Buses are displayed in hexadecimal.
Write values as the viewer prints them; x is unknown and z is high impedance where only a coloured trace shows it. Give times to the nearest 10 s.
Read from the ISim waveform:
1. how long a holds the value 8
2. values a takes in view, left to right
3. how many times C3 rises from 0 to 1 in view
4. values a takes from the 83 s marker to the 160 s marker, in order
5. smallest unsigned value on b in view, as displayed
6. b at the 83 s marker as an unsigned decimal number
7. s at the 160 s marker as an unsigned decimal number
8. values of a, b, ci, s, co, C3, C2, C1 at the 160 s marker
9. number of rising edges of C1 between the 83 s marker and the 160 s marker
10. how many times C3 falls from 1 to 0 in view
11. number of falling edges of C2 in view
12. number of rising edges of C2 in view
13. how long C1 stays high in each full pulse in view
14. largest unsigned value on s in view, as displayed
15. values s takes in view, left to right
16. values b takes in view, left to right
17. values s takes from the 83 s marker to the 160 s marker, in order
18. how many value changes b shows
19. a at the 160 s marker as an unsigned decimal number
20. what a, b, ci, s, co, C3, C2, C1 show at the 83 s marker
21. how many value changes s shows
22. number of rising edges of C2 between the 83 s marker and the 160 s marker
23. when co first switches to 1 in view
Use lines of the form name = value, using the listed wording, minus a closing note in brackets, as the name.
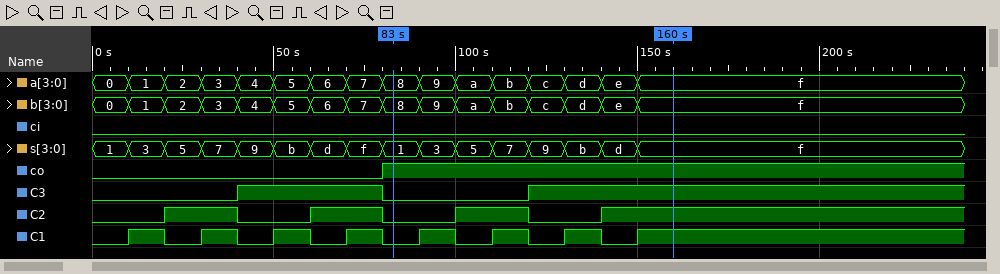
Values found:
how long a holds the value 8 = 10 s
values a takes in view, left to right = 0, 1, 2, 3, 4, 5, 6, 7, 8, 9, a, b, c, d, e, f
how many times C3 rises from 0 to 1 in view = 2
values a takes from the 83 s marker to the 160 s marker, in order = 8, 9, a, b, c, d, e, f
smallest unsigned value on b in view, as displayed = 0
b at the 83 s marker as an unsigned decimal number = 8
s at the 160 s marker as an unsigned decimal number = 15
values of a, b, ci, s, co, C3, C2, C1 at the 160 s marker = a=f, b=f, ci=0, s=f, co=1, C3=1, C2=1, C1=1
number of rising edges of C1 between the 83 s marker and the 160 s marker = 4
how many times C3 falls from 1 to 0 in view = 1
number of falling edges of C2 in view = 3
number of rising edges of C2 in view = 4
how long C1 stays high in each full pulse in view = 10 s, 10 s, 10 s, 10 s, 10 s, 10 s, 10 s
largest unsigned value on s in view, as displayed = f
values s takes in view, left to right = 1, 3, 5, 7, 9, b, d, f, 1, 3, 5, 7, 9, b, d, f
values b takes in view, left to right = 0, 1, 2, 3, 4, 5, 6, 7, 8, 9, a, b, c, d, e, f
values s takes from the 83 s marker to the 160 s marker, in order = 1, 3, 5, 7, 9, b, d, f
how many value changes b shows = 15
a at the 160 s marker as an unsigned decimal number = 15
what a, b, ci, s, co, C3, C2, C1 show at the 83 s marker = a=8, b=8, ci=0, s=1, co=1, C3=0, C2=0, C1=0
how many value changes s shows = 15
number of rising edges of C2 between the 83 s marker and the 160 s marker = 2
when co first switches to 1 in view = 80 s
